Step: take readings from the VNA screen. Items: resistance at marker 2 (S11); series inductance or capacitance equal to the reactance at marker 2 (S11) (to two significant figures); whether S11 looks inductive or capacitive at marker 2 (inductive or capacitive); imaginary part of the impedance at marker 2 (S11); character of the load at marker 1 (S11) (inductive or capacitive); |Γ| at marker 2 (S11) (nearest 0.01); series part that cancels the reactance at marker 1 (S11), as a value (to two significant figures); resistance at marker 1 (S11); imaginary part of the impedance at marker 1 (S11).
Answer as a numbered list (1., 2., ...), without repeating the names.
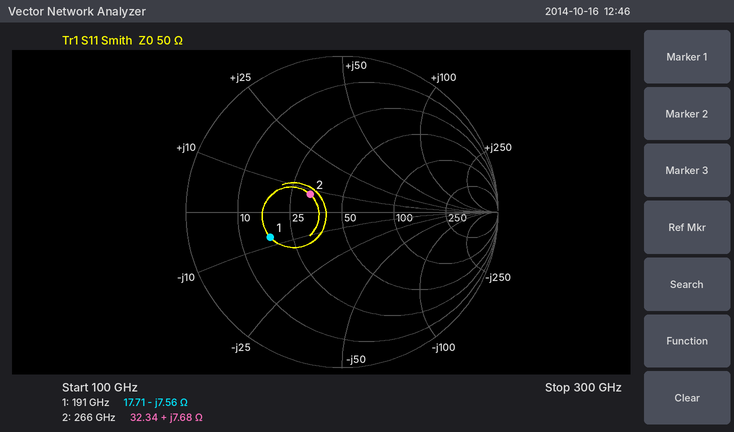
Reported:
1. 32.34 Ω
2. 4.6 pH
3. inductive
4. +7.68 Ω
5. capacitive
6. 0.23
7. 6.3 pH
8. 17.71 Ω
9. -7.56 Ω
